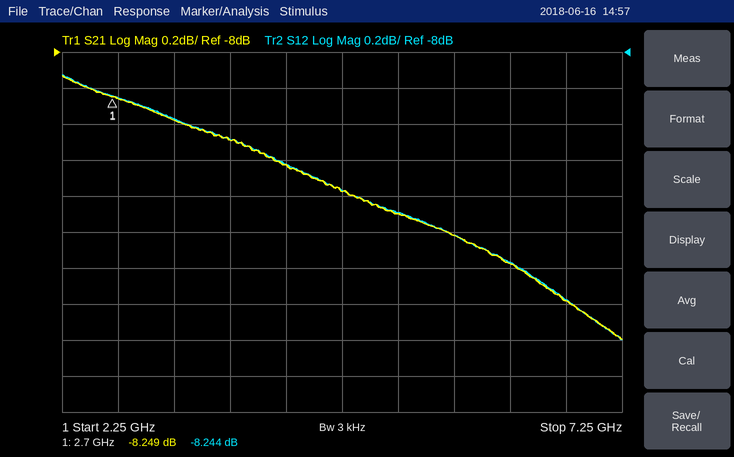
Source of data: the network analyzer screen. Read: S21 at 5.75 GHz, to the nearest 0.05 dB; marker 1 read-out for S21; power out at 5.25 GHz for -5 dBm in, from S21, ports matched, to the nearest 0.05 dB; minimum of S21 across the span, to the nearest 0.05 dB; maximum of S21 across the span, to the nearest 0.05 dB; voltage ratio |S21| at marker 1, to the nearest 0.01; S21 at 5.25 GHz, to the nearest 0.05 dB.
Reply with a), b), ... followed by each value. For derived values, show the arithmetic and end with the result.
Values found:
a) -9.00 dB
b) -8.249 dB
c) -5 dBm + (-8.90 dB) = -13.90 dBm
d) -9.60 dB
e) -8.15 dB
f) 10^(-8.249/20) ≈ 0.39
g) -8.90 dB
